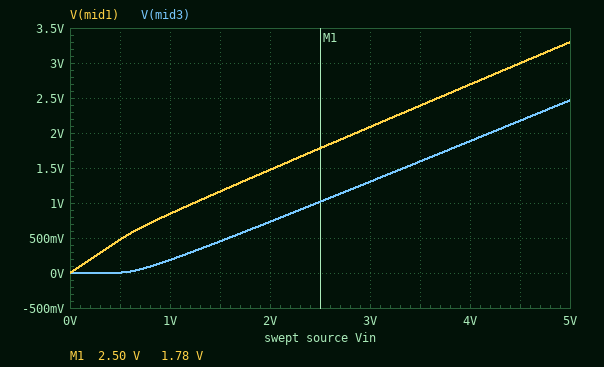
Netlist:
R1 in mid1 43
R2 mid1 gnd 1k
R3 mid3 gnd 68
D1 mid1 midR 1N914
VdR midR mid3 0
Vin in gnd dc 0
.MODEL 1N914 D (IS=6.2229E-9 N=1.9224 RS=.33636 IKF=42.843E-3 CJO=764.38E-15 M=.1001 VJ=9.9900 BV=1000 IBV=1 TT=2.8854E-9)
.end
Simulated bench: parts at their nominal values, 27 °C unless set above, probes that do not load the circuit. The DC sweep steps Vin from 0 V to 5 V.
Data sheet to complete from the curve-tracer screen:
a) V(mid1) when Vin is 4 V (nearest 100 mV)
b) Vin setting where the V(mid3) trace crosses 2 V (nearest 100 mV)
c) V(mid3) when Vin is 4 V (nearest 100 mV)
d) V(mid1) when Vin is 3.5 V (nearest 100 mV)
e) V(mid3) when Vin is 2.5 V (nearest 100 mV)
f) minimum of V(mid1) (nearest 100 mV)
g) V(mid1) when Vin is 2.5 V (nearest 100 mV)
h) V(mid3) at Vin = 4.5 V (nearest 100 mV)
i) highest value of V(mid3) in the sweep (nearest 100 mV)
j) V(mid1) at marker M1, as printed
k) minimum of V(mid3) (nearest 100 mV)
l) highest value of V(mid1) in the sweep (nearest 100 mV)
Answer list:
2.7 V
4.2 V
1.9 V
2.4 V
1.0 V
0 V
1.8 V
2.2 V
2.5 V
1.78 V
0 V
3.3 V
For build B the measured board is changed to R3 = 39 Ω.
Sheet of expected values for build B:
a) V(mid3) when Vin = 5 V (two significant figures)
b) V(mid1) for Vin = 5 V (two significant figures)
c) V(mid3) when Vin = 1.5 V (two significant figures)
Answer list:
1.9 V
2.8 V
340 mV
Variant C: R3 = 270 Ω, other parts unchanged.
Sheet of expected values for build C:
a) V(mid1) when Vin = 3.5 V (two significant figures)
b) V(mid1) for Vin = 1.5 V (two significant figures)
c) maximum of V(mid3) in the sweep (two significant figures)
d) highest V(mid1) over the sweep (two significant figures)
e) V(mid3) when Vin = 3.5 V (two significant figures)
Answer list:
3.0 V
1.3 V
3.5 V
4.3 V
2.3 V
